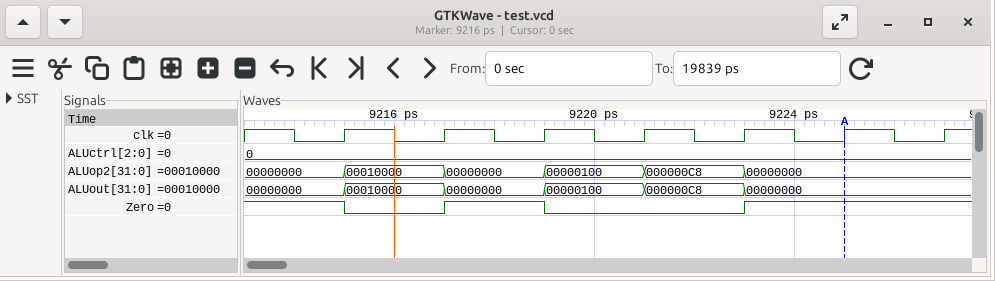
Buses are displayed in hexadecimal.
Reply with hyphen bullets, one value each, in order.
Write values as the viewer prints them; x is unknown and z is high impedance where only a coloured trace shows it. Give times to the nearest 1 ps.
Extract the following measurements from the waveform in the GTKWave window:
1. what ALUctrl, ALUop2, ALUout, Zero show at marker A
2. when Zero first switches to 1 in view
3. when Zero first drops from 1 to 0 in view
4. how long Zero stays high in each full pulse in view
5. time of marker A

- ALUctrl=0, ALUop2=00000000, ALUout=00000000, Zero=1
- 9217 ps
- 9215 ps
- 2 ps
- 9225 ps
